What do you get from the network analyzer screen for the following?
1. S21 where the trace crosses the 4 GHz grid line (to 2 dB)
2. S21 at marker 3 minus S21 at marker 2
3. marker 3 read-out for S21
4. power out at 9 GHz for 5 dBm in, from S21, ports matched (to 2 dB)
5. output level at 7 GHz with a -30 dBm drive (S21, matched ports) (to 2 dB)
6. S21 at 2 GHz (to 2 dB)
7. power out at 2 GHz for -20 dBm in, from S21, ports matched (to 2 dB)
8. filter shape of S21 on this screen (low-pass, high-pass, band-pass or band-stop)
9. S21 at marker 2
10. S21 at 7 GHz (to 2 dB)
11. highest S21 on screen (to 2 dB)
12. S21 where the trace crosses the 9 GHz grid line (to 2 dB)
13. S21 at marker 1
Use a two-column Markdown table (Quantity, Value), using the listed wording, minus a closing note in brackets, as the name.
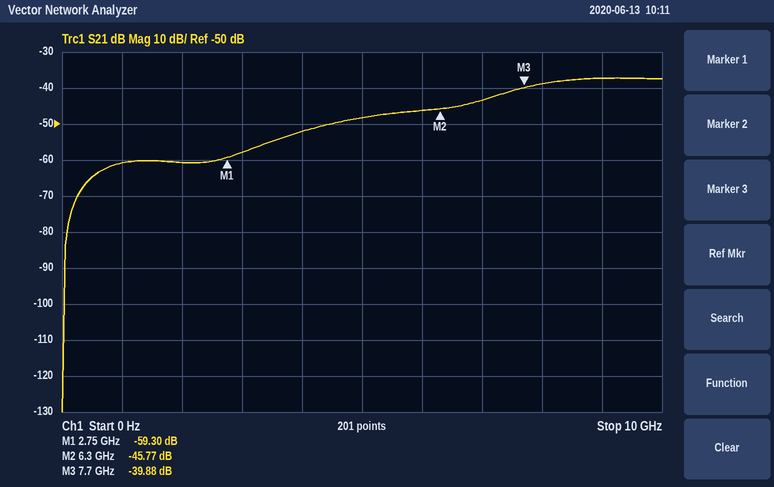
| Quantity | Value |
|---|---|
| S21 where the trace crosses the 4 GHz grid line | -52 dB |
| S21 at marker 3 minus S21 at marker 2 | 5.89 dB |
| marker 3 read-out for S21 | -39.88 dB |
| power out at 9 GHz for 5 dBm in, from S21, ports matched | -32 dBm |
| output level at 7 GHz with a -30 dBm drive (S21, matched ports) | -74 dBm |
| S21 at 2 GHz | -60 dB |
| power out at 2 GHz for -20 dBm in, from S21, ports matched | -80 dBm |
| filter shape of S21 on this screen | high-pass |
| S21 at marker 2 | -45.77 dB |
| S21 at 7 GHz | -44 dB |
| highest S21 on screen | -38 dB |
| S21 where the trace crosses the 9 GHz grid line | -38 dB |
| S21 at marker 1 | -59.30 dB |
